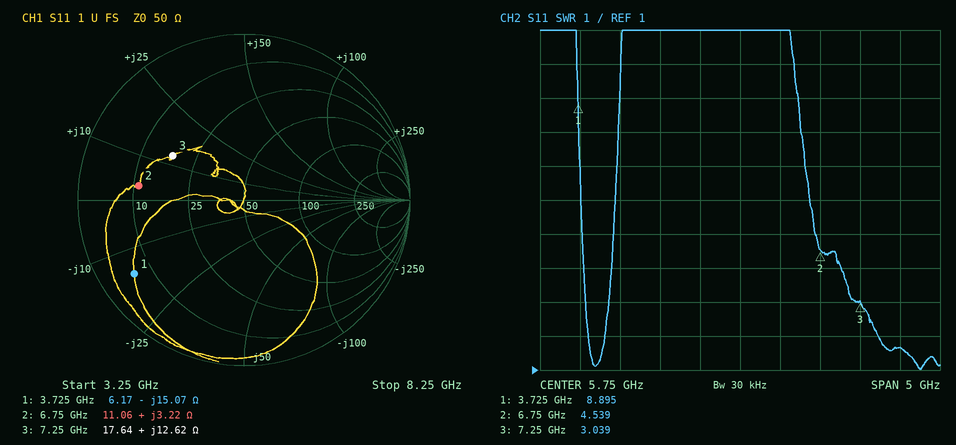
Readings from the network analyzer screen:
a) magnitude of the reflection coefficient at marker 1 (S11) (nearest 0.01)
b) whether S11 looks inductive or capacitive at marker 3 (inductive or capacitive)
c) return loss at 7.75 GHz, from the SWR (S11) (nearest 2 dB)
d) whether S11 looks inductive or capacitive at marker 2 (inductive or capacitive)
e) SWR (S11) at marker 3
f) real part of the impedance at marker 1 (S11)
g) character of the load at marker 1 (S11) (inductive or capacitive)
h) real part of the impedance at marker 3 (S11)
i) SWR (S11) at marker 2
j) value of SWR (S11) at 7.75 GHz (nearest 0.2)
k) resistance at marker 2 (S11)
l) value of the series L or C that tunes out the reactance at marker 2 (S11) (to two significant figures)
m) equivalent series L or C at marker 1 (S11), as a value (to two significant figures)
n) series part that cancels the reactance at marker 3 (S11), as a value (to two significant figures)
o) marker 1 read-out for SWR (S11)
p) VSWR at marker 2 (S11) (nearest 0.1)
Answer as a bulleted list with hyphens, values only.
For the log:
- 0.80
- inductive
- 12 dB
- inductive
- 3.039
- 6.17 Ω
- capacitive
- 17.64 Ω
- 4.539
- 1.6
- 11.06 Ω
- 7.3 pF
- 2.8 pF
- 1.7 pF
- 8.895
- 4.5
